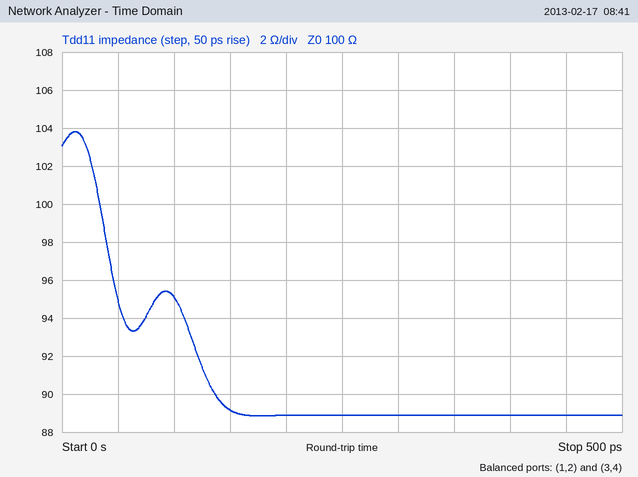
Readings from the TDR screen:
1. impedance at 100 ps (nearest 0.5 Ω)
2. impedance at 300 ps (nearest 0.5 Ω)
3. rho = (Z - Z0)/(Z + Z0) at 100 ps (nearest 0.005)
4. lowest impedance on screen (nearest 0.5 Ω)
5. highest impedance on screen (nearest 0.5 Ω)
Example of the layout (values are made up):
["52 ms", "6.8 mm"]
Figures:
["95.0 Ω", "89.0 Ω", "-0.025", "89.0 Ω", "104.0 Ω"]
